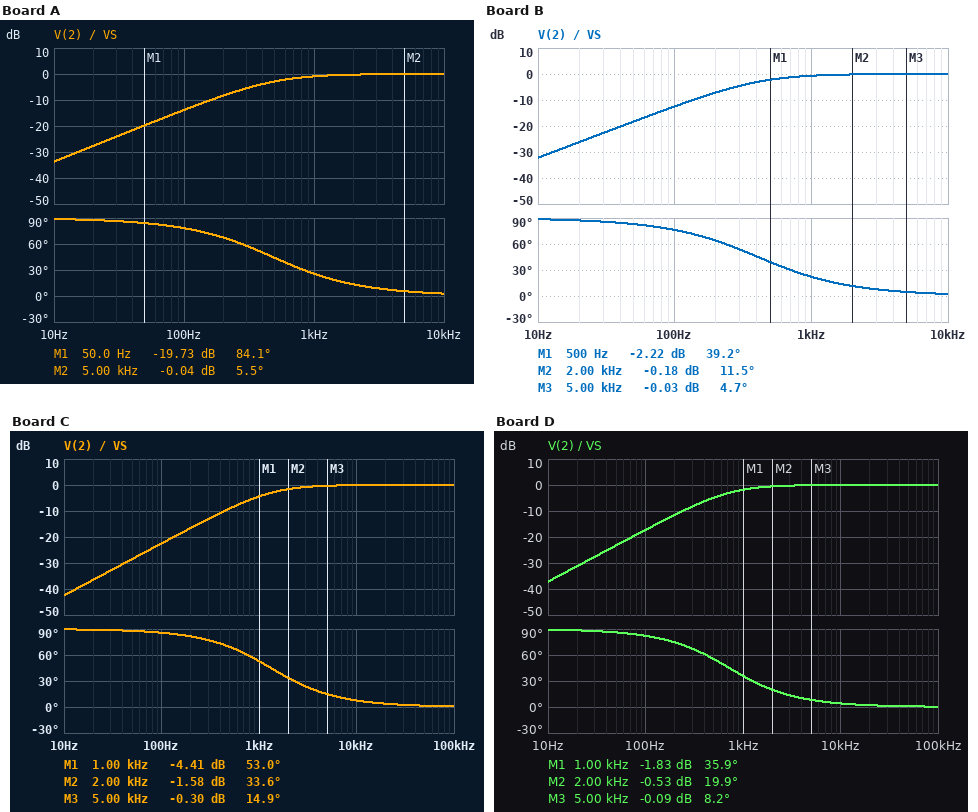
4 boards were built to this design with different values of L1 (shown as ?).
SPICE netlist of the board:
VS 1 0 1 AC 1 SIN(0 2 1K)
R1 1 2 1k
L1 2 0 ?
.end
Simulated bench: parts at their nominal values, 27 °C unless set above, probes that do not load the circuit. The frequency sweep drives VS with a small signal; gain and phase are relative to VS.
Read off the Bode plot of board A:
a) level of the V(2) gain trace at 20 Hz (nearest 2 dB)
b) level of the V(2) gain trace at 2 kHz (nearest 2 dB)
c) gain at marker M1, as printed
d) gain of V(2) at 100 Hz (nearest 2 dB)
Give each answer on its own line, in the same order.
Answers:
-28 dB
0 dB
-19.73 dB
-14 dB
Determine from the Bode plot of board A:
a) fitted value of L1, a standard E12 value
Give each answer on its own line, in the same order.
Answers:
330 mH
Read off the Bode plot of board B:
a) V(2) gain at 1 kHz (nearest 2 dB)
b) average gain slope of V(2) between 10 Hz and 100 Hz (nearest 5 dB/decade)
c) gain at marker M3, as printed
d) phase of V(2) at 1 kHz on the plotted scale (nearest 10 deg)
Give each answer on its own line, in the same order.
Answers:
0 dB
20 dB/decade
-0.03 dB
20 deg
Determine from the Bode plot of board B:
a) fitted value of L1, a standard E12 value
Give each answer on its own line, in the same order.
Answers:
390 mH
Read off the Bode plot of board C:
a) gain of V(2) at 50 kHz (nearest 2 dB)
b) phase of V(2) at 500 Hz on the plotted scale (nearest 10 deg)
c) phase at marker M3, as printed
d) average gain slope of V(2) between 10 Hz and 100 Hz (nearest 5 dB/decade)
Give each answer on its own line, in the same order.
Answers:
0 dB
70 deg
14.9 deg
20 dB/decade
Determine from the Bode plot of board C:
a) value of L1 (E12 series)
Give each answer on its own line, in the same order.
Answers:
120 mH
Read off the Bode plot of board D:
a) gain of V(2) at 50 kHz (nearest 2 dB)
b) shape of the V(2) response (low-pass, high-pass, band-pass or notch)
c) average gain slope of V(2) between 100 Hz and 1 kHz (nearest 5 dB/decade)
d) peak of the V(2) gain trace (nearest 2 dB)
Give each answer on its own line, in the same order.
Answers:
0 dB
high-pass
15 dB/decade
0 dB
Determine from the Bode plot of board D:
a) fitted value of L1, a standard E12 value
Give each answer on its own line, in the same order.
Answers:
220 mH
